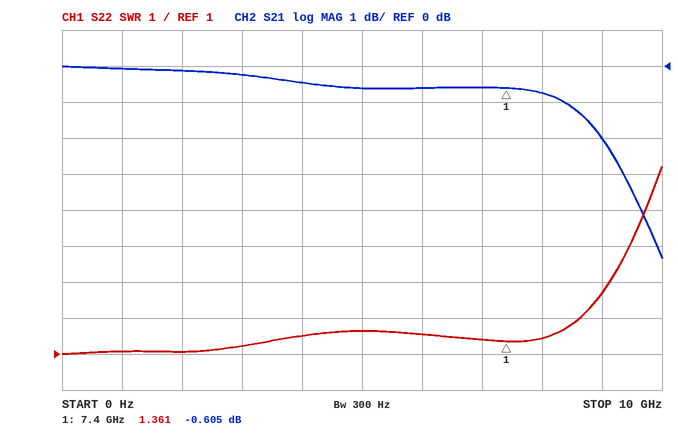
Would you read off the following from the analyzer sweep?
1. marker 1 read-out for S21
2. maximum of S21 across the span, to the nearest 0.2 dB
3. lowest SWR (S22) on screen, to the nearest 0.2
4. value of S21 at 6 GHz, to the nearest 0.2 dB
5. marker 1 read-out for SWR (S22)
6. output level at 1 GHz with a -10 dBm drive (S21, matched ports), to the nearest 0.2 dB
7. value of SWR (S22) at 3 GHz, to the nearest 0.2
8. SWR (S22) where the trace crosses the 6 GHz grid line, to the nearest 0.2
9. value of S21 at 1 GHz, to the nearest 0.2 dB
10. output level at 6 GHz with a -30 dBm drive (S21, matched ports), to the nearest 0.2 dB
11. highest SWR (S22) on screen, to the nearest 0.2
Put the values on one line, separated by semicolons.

-0.605 dB; 0.0 dB; 1.0; -0.6 dB; 1.361; -10.0 dBm; 1.2; 1.6; 0.0 dB; -30.6 dBm; 6.2
